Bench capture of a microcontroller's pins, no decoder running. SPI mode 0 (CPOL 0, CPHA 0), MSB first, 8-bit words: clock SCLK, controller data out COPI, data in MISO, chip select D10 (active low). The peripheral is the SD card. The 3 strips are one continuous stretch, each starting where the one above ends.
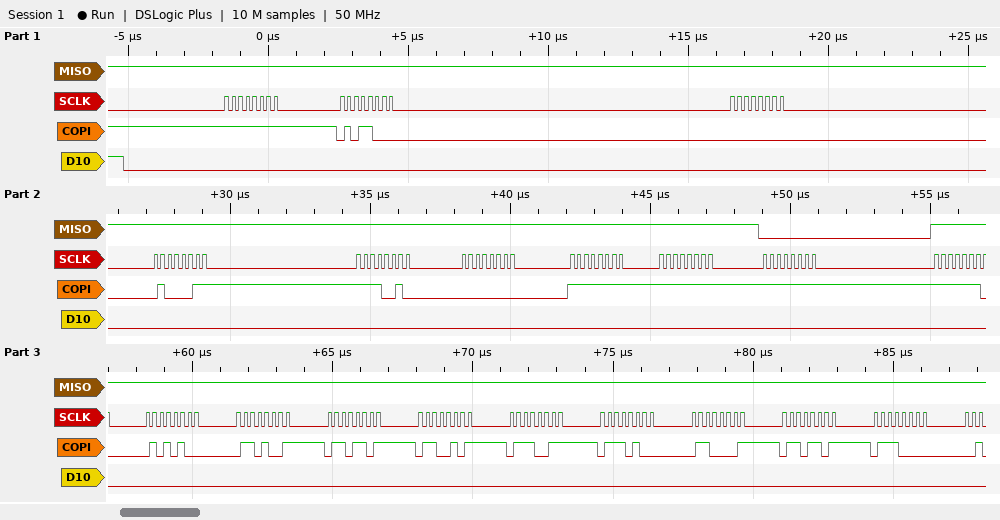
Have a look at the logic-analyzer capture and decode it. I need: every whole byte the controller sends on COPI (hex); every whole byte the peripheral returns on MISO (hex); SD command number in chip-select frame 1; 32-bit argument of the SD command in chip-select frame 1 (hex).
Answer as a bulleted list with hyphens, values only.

- 0xFF 0x58 0x00 0x43 0xF2 0x00 0xFF 0xFF 0xFF 0xFE 0x54 0x69 0x6D 0x65 0x73 0x74 0x61 0x6D 0x70
- 0xFF 0xFF 0xFF 0xFF 0xFF 0xFF 0xFF 0xFF 0x00 0xFF 0xFF 0xFF 0xFF 0xFF 0xFF 0xFF 0xFF 0xFF 0xFF
- CMD24
- 0x0043F200
